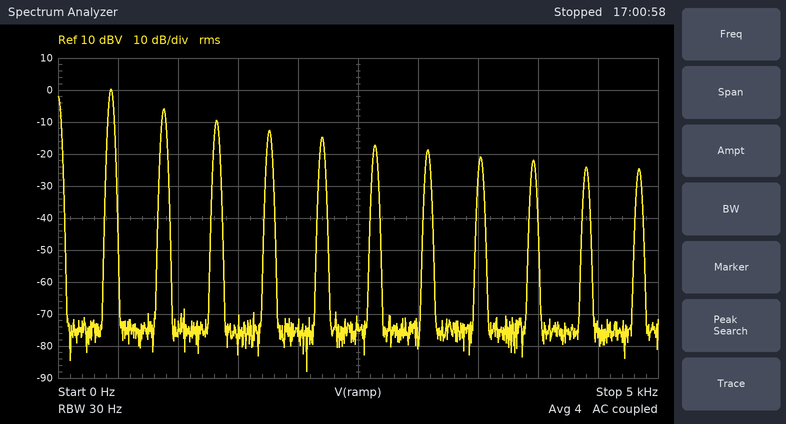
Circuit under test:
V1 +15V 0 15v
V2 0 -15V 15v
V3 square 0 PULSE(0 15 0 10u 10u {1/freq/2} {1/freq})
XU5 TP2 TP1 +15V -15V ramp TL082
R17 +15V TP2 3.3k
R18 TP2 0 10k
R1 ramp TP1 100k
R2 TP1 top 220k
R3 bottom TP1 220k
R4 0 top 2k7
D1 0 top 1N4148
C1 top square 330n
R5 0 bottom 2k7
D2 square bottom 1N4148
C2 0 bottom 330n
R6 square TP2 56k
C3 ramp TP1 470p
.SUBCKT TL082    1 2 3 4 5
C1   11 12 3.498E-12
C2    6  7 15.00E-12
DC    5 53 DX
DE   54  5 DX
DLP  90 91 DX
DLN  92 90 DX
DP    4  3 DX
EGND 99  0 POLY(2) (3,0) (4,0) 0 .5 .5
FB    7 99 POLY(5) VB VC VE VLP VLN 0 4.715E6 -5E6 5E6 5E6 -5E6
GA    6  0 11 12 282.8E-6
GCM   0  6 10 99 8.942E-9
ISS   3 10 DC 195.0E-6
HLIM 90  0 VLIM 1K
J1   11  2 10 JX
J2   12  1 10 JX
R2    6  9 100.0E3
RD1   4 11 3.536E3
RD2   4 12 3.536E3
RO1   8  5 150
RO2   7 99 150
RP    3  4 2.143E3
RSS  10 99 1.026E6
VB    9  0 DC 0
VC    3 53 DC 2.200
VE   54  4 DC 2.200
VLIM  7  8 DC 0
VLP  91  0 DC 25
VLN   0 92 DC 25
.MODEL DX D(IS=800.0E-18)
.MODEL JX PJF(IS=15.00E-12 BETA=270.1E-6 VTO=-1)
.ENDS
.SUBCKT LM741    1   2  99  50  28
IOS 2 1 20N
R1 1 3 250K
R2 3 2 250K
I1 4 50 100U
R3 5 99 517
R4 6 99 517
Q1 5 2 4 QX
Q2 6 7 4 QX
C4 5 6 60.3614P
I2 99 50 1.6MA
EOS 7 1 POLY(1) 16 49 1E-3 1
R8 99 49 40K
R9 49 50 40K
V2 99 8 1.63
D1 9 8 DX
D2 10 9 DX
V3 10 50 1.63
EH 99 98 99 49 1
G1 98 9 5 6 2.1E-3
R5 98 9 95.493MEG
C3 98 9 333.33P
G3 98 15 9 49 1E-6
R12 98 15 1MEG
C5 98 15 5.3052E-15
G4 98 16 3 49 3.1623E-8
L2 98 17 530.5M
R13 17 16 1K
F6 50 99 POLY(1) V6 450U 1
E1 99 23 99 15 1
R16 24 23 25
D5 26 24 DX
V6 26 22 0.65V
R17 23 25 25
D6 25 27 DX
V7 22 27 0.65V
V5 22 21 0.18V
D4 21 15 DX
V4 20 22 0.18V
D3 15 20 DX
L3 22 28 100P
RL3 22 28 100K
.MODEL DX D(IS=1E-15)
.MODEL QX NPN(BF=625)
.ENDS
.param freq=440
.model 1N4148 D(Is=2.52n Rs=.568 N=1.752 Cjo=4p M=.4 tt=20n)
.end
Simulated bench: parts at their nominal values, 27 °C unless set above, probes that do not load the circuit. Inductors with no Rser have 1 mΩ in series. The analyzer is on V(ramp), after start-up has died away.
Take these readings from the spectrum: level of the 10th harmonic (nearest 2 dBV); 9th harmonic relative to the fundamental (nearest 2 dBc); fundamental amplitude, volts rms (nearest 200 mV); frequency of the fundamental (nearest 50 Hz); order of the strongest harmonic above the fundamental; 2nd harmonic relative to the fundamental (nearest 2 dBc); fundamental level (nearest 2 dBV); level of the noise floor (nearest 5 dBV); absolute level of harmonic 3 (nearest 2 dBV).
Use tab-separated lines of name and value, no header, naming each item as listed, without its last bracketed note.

level of the 10th harmonic	-24 dBV
9th harmonic relative to the fundamental	-22 dBc
fundamental amplitude, volts rms	1.0 V
frequency of the fundamental	450 Hz
order of the strongest harmonic above the fundamental	2
2nd harmonic relative to the fundamental	-6 dBc
fundamental level	0 dBV
level of the noise floor	-75 dBV
absolute level of harmonic 3	-10 dBV
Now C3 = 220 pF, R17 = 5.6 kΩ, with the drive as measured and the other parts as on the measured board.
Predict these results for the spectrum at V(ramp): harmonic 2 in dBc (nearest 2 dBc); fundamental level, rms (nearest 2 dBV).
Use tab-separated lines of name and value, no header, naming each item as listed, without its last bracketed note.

harmonic 2 in dBc	-8 dBc
fundamental level, rms	6 dBV
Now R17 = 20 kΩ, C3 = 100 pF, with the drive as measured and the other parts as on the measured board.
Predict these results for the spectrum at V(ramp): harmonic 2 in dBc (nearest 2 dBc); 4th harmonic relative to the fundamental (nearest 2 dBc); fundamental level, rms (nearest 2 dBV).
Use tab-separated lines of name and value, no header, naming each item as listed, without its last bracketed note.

harmonic 2 in dBc	-4 dBc
4th harmonic relative to the fundamental	-10 dBc
fundamental level, rms	4 dBV
